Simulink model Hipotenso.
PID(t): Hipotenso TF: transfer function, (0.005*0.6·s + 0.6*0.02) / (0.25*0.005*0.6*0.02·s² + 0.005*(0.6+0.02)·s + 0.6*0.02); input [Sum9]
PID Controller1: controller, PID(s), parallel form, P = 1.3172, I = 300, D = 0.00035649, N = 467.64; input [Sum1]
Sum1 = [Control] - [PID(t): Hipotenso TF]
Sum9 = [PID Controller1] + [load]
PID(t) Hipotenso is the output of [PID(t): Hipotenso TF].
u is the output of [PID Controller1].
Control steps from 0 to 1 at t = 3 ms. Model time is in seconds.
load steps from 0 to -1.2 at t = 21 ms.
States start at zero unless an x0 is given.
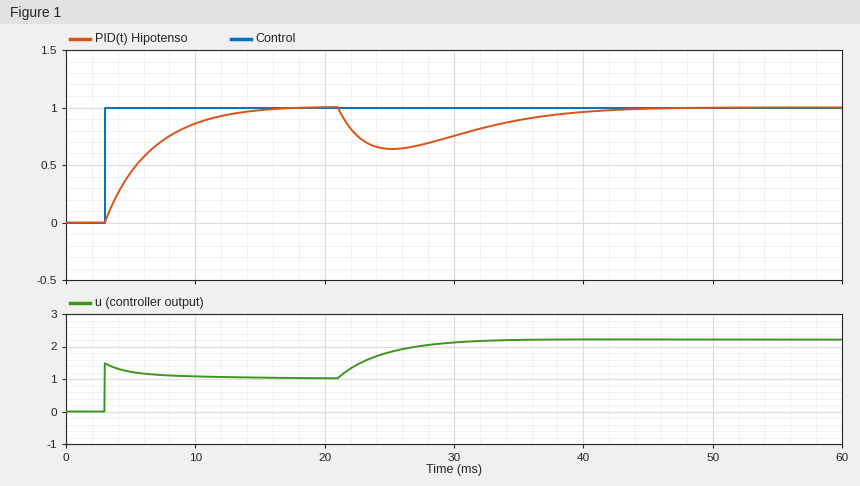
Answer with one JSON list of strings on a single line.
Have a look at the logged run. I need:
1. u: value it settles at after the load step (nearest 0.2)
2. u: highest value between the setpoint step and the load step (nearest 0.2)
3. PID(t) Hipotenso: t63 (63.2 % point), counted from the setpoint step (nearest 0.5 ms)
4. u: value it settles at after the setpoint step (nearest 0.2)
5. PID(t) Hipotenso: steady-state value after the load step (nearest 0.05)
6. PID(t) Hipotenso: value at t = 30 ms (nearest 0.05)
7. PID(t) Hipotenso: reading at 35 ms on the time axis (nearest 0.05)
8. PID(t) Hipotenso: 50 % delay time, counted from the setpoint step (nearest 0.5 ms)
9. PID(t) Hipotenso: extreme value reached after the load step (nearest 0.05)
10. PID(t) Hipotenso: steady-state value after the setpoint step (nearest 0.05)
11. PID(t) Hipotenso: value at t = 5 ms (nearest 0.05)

["2.2", "1.4", "3.5 ms", "1.0", "1.00", "0.75", "0.90", "2.5 ms", "0.65", "1.00", "0.45"]
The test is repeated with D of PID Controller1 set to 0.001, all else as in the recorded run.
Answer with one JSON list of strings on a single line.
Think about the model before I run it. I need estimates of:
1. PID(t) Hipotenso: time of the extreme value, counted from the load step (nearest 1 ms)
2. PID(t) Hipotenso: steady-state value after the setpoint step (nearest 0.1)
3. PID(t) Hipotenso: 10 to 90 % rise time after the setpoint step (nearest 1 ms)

["4 ms", "1.0", "8 ms"]
